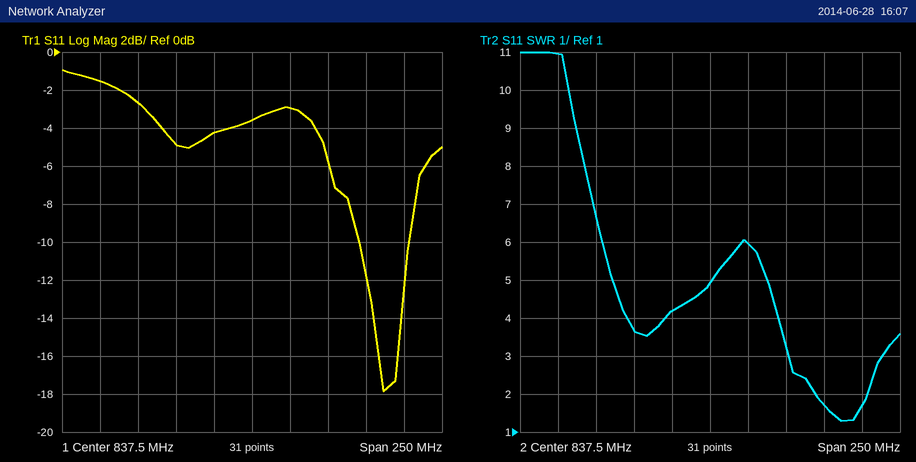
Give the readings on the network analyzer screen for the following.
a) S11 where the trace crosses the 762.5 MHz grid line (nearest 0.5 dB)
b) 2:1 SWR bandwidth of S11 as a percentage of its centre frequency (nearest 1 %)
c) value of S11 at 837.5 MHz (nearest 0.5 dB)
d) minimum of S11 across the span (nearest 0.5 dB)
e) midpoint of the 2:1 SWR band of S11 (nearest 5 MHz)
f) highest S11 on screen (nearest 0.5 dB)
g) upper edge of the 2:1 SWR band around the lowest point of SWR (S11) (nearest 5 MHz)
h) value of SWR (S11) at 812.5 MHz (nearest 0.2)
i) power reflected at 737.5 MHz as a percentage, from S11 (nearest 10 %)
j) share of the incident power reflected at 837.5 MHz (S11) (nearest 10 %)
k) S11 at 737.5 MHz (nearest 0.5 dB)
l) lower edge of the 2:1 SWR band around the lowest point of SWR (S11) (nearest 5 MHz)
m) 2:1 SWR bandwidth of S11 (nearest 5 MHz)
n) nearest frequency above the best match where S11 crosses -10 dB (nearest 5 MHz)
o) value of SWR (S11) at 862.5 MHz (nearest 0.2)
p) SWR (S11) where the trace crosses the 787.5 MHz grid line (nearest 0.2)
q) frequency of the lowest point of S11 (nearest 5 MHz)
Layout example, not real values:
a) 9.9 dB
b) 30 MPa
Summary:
a) -2.5 dB
b) 4 %
c) -3.5 dB
d) -18.0 dB
e) 925 MHz
f) -1.0 dB
g) 940 MHz
h) 4.2
i) 70 %
j) 40 %
k) -1.5 dB
l) 905 MHz
m) 35 MHz
n) 940 MHz
o) 6.0
p) 3.6
q) 925 MHz
